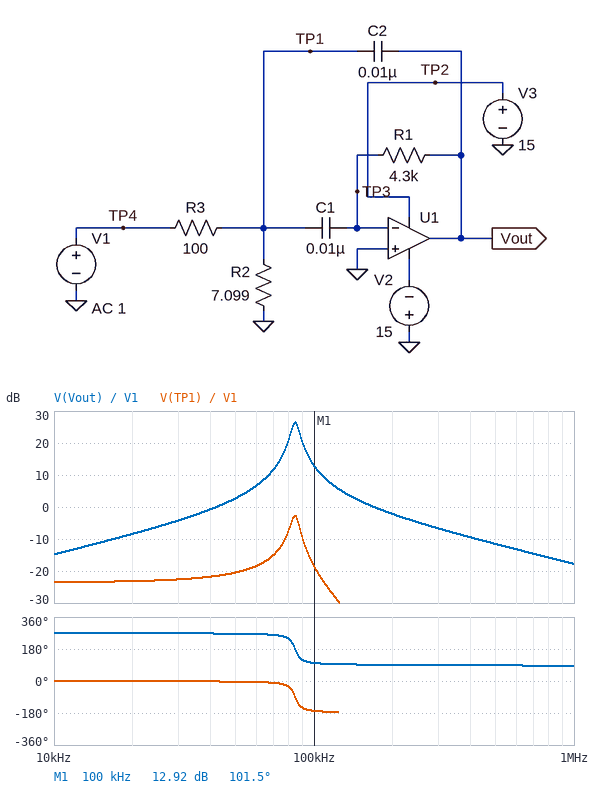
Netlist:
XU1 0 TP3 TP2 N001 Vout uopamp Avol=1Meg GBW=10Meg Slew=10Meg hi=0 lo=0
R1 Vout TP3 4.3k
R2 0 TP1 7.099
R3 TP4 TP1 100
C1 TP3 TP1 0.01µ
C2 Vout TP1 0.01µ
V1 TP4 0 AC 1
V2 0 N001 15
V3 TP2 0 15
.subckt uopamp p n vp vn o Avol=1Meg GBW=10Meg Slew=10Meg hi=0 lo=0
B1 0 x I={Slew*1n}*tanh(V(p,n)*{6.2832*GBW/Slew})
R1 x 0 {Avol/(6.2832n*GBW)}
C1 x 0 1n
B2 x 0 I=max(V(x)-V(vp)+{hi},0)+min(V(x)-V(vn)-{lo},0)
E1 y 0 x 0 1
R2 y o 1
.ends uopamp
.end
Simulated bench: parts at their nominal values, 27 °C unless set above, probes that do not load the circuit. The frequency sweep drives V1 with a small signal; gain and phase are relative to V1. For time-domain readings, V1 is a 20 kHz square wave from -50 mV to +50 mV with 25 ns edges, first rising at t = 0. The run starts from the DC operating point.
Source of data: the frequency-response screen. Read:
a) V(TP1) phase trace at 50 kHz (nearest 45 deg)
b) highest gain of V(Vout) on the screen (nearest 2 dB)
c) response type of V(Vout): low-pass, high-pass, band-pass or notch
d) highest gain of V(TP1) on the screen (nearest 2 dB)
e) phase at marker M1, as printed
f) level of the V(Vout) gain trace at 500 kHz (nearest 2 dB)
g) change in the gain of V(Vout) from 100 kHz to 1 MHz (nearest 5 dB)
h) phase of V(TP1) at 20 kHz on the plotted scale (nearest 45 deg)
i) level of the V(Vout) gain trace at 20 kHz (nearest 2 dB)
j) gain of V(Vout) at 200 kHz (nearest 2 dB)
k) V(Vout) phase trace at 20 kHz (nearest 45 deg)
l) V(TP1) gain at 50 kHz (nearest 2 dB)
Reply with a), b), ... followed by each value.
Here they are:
a) 0 deg
b) 26 dB
c) band-pass
d) -2 dB
e) 101.5 deg
f) -12 dB
g) -30 dB
h) 0 deg
i) -8 dB
j) -2 dB
k) 270 deg
l) -20 dB
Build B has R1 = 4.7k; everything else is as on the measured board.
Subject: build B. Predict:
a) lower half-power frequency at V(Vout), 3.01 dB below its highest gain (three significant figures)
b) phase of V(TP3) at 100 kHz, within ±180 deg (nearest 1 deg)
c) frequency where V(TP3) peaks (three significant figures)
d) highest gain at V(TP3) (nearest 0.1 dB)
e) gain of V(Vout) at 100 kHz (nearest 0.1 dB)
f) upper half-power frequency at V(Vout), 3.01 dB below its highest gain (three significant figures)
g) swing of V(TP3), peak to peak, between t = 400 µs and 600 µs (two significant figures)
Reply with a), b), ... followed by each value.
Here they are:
a) 78.3 kHz
b) 9 deg
c) 81.1 kHz
d) -14.5 dB
e) 11.3 dB
f) 83.8 kHz
g) 1.6 mV
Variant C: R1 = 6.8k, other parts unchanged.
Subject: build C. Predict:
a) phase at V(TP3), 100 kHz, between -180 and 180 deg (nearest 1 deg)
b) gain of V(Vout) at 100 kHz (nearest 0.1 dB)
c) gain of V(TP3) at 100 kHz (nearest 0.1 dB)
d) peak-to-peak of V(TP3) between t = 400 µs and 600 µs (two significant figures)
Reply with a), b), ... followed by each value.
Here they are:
a) 4 deg
b) 7.4 dB
c) -32.6 dB
d) 2.5 mV
